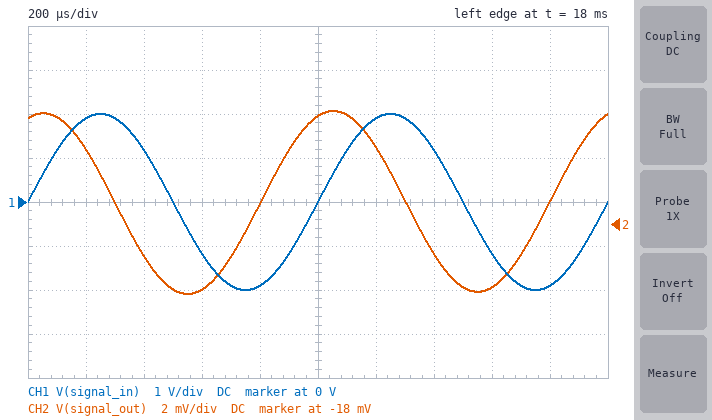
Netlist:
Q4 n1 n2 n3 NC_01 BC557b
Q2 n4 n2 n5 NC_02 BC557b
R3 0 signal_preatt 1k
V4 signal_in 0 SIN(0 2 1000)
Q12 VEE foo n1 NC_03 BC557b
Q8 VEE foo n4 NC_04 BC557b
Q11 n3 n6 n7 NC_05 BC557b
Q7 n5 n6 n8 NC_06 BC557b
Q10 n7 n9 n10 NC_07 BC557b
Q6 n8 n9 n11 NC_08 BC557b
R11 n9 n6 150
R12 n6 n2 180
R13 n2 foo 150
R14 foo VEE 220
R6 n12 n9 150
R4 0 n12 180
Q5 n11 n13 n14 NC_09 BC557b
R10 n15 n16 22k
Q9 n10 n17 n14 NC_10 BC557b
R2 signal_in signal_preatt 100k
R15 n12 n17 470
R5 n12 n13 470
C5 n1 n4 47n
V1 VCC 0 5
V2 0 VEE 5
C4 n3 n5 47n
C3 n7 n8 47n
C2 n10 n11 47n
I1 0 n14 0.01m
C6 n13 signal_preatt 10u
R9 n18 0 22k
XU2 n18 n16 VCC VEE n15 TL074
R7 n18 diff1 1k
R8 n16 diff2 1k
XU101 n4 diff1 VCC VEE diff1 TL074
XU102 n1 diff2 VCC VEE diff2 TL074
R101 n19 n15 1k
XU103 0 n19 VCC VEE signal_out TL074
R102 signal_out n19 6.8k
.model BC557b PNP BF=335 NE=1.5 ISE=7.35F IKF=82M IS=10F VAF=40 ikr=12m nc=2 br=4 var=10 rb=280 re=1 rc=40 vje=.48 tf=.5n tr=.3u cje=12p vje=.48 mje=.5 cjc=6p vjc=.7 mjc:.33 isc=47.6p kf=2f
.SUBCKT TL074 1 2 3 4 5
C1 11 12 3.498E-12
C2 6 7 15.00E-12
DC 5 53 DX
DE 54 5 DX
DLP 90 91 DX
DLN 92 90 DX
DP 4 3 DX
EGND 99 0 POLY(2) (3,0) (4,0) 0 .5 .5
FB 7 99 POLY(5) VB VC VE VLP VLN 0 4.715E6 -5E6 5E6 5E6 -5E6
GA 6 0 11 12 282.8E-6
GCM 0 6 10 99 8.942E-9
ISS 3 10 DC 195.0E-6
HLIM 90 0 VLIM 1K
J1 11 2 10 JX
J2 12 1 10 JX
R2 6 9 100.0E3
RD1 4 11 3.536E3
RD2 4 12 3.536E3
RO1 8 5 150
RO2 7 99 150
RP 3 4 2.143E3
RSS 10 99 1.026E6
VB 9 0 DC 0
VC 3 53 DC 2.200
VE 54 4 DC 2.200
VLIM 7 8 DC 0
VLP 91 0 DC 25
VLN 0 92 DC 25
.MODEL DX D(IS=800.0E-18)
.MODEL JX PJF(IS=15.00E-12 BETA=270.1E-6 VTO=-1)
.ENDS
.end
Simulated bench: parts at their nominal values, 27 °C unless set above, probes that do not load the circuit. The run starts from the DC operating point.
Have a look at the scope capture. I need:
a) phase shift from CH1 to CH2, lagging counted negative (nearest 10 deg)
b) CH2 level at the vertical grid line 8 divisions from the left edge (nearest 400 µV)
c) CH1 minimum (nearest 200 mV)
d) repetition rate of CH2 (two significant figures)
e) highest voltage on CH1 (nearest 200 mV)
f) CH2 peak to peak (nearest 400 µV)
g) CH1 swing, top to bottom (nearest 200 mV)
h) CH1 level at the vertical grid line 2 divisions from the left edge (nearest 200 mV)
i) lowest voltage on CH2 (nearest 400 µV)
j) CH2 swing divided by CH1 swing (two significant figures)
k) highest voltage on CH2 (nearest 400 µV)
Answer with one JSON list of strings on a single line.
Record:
["70 deg", "-20.8 mV", "-2.0 V", "1.0 kHz", "2.0 V", "8.4 mV", "4.0 V", "1.2 V", "-21.2 mV", "0.0021", "-12.8 mV"]
